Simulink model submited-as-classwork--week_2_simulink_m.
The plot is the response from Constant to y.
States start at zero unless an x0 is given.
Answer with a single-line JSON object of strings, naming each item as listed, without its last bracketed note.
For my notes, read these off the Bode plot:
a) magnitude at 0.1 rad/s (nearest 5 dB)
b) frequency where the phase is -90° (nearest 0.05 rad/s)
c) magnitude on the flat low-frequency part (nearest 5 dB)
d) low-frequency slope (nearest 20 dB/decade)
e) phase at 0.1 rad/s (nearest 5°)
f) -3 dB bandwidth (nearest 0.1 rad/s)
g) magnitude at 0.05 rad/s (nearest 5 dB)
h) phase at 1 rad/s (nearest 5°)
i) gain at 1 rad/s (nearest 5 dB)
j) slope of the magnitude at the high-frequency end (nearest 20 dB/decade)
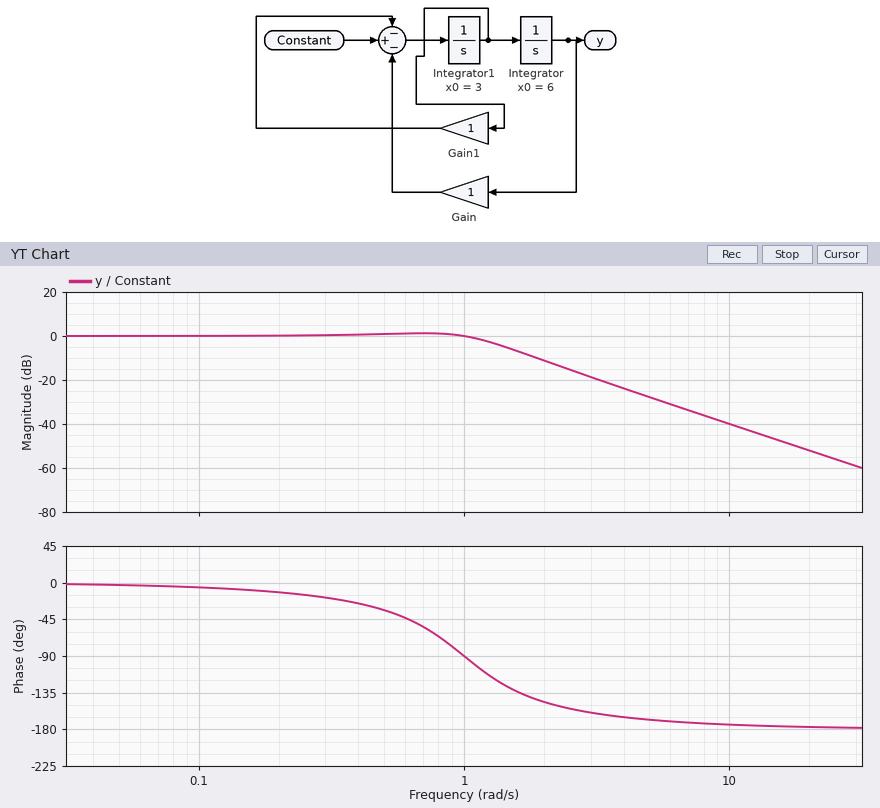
{"magnitude at 0.1 rad/s": "0 dB", "frequency where the phase is -90°": "1.00 rad/s", "magnitude on the flat low-frequency part": "0 dB", "low-frequency slope": "0 dB/decade", "phase at 0.1 rad/s": "-5°", "-3 dB bandwidth": "1.3 rad/s", "magnitude at 0.05 rad/s": "0 dB", "phase at 1 rad/s": "-90°", "gain at 1 rad/s": "0 dB", "slope of the magnitude at the high-frequency end": "-40 dB/decade"}
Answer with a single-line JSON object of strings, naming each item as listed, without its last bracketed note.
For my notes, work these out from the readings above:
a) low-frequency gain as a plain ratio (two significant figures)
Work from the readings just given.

{"low-frequency gain as a plain ratio": "1.0"}
